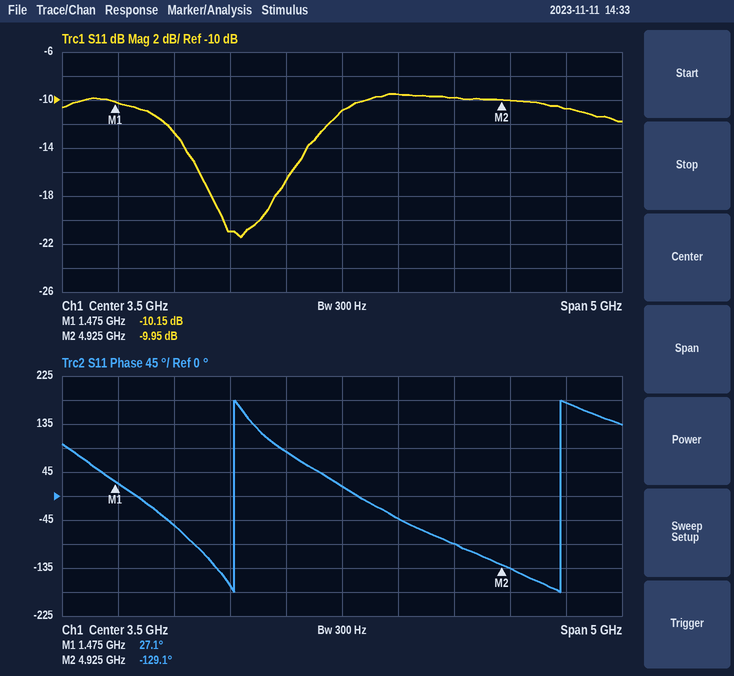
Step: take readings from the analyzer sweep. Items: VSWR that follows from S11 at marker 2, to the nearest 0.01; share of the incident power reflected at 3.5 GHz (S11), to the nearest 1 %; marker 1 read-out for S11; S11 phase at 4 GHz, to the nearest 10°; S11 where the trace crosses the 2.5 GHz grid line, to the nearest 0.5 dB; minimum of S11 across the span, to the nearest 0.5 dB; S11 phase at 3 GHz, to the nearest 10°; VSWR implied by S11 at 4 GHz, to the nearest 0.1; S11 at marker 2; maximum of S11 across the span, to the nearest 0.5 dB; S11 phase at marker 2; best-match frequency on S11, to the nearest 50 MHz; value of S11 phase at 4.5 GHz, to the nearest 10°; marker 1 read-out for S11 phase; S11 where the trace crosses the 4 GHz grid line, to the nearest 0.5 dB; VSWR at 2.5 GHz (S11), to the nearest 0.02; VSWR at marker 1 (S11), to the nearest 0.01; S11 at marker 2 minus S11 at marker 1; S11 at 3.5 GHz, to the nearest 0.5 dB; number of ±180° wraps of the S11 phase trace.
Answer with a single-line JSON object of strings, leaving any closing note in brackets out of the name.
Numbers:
{"VSWR that follows from S11 at marker 2, to the nearest 0.01": "1.93", "share of the incident power reflected at 3.5 GHz (S11), to the nearest 1 %": "8 %", "marker 1 read-out for S11": "-10.15 dB", "S11 phase at 4 GHz, to the nearest 10°": "-40°", "S11 where the trace crosses the 2.5 GHz grid line, to the nearest 0.5 dB": "-21.0 dB", "minimum of S11 across the span, to the nearest 0.5 dB": "-21.5 dB", "S11 phase at 3 GHz, to the nearest 10°": "80°", "VSWR implied by S11 at 4 GHz, to the nearest 0.1": "2.0", "S11 at marker 2": "-9.95 dB", "maximum of S11 across the span, to the nearest 0.5 dB": "-9.5 dB", "S11 phase at marker 2": "-129.1°", "best-match frequency on S11, to the nearest 50 MHz": "2.60 GHz", "value of S11 phase at 4.5 GHz, to the nearest 10°": "-90°", "marker 1 read-out for S11 phase": "27.1°", "S11 where the trace crosses the 4 GHz grid line, to the nearest 0.5 dB": "-9.5 dB", "VSWR at 2.5 GHz (S11), to the nearest 0.02": "1.20", "VSWR at marker 1 (S11), to the nearest 0.01": "1.90", "S11 at marker 2 minus S11 at marker 1": "0.20 dB", "S11 at 3.5 GHz, to the nearest 0.5 dB": "-11.0 dB", "number of ±180° wraps of the S11 phase trace": "2"}
